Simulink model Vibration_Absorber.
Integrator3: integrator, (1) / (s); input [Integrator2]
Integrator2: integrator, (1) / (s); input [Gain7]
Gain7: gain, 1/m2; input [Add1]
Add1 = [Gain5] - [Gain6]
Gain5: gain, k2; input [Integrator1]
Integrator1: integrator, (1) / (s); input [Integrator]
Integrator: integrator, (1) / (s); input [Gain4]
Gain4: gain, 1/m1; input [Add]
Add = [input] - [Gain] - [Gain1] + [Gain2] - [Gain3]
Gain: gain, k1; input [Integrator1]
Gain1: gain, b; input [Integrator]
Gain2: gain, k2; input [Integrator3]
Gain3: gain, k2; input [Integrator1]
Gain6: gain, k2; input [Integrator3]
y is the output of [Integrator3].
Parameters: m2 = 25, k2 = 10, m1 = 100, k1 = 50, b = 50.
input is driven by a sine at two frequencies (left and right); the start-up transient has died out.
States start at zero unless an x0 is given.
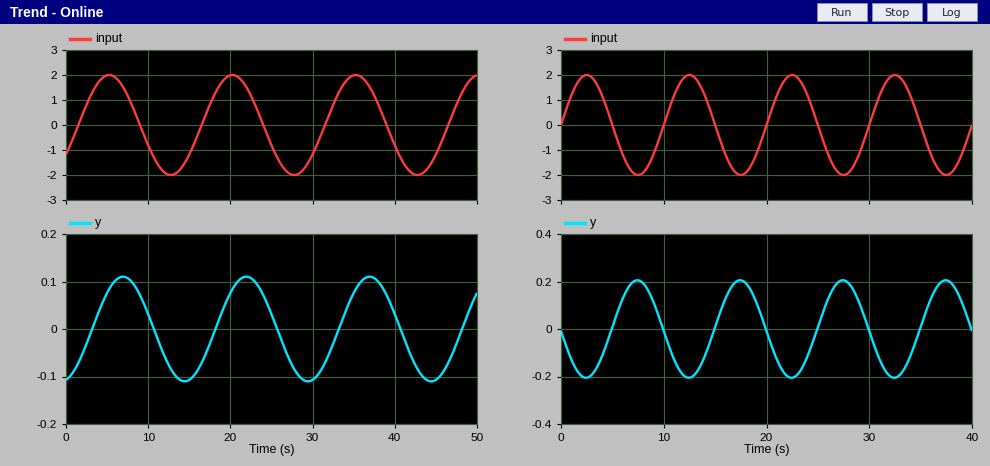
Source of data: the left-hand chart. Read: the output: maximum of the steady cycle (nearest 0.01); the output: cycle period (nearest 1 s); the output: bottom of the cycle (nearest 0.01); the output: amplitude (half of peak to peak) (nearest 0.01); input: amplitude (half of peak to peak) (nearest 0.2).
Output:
0.11
15 s
-0.11
0.11
2.0
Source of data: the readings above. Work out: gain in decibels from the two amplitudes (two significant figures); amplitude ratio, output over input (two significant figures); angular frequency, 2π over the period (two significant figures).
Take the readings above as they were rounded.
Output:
-25 dB
0.055
0.42 rad/s
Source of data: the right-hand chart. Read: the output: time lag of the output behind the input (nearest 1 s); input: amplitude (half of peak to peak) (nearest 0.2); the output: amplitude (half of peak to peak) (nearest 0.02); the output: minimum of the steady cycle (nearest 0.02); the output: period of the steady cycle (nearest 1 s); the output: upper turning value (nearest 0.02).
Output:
5 s
2.0
0.20
-0.20
10 s
0.20
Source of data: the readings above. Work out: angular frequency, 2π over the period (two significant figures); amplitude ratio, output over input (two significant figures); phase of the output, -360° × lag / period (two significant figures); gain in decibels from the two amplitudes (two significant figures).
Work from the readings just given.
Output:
0.63 rad/s
0.10
-180°
-20 dB
